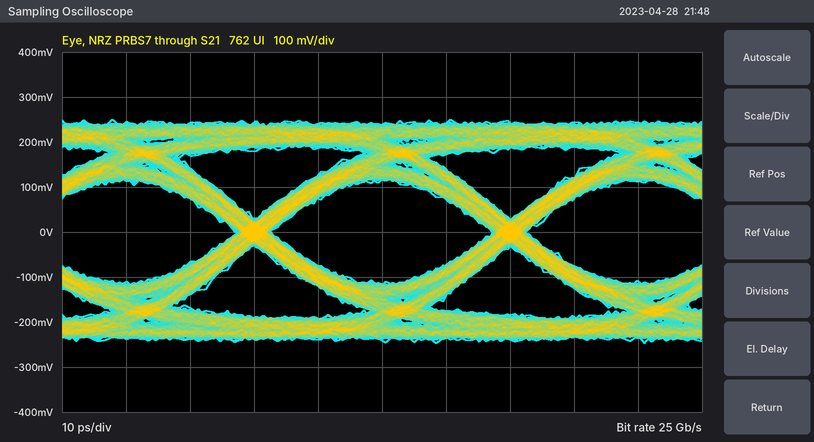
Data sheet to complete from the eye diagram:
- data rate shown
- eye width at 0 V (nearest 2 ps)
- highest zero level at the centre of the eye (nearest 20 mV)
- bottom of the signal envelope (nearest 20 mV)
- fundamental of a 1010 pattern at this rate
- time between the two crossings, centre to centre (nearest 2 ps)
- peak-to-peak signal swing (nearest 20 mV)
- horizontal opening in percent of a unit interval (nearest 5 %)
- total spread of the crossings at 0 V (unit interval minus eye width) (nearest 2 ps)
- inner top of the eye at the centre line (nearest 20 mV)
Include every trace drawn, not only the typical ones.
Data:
25 Gb/s
34 ps
-120 mV
-240 mV
12.5 GHz
40 ps
500 mV
85 %
6 ps
120 mV
